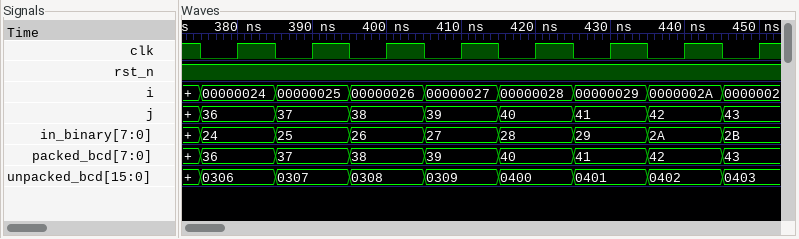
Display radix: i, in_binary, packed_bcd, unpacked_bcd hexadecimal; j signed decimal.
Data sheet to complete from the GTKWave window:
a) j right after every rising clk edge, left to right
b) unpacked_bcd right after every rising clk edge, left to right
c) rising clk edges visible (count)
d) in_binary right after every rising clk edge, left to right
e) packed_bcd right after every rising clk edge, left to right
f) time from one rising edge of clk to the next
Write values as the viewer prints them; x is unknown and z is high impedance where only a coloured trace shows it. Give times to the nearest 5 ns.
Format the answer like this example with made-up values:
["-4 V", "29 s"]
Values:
["36, 37, 38, 39, 40, 41, 42, 43", "0306, 0307, 0308, 0309, 0400, 0401, 0402, 0403", "8", "24, 25, 26, 27, 28, 29, 2A, 2B", "36, 37, 38, 39, 40, 41, 42, 43", "10 ns"]
